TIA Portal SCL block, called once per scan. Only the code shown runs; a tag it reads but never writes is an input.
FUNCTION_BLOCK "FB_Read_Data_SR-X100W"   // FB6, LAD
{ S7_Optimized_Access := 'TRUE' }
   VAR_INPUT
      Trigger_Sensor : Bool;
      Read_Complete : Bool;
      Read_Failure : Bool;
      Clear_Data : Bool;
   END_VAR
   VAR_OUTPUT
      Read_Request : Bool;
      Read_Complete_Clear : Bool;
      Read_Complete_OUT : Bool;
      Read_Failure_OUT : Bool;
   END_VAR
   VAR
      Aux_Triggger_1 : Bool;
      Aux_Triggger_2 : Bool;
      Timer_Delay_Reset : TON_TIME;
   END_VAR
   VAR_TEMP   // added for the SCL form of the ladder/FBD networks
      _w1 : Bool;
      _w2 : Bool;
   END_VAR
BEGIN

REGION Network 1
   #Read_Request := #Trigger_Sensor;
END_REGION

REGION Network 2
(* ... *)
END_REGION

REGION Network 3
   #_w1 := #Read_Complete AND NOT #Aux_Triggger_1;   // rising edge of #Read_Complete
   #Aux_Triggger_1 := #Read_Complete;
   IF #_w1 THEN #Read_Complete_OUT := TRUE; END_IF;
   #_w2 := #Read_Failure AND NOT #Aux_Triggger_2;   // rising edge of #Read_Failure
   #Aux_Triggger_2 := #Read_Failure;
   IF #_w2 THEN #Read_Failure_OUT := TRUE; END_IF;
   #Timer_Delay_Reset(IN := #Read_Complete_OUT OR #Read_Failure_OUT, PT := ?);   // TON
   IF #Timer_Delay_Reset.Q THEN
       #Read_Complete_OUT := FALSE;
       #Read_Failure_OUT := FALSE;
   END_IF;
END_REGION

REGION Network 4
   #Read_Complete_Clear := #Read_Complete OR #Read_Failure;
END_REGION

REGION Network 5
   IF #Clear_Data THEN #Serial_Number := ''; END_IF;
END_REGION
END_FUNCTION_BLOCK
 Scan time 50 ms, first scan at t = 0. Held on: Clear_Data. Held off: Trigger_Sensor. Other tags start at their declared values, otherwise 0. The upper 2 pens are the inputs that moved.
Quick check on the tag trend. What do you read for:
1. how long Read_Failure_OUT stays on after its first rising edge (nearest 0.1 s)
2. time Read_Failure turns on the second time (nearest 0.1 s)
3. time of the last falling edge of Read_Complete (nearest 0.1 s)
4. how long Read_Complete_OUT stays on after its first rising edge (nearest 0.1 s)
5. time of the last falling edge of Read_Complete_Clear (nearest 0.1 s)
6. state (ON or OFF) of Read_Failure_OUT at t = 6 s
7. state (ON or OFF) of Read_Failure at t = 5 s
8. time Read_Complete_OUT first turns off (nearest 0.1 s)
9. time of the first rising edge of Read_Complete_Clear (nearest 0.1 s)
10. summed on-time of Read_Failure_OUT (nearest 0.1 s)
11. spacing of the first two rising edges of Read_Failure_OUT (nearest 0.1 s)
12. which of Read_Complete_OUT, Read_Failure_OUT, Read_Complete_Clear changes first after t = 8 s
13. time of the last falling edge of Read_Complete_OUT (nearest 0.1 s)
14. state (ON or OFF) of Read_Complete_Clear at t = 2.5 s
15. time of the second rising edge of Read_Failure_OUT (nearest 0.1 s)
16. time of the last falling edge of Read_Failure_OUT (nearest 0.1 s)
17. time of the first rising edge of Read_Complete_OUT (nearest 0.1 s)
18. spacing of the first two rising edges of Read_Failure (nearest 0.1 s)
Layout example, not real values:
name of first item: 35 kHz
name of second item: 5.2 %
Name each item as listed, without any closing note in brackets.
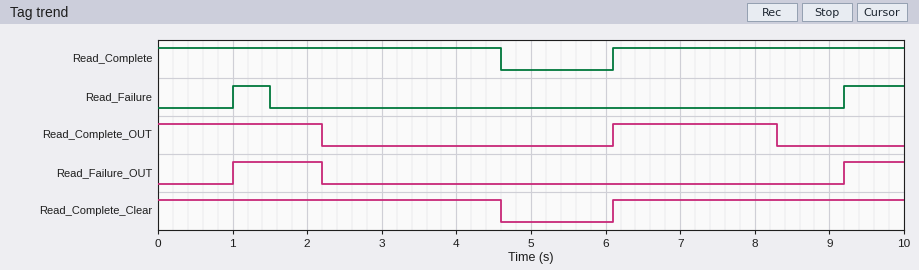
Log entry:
how long Read_Failure_OUT stays on after its first rising edge: 1.2 s
time Read_Failure turns on the second time: 9.2 s
time of the last falling edge of Read_Complete: 4.6 s
how long Read_Complete_OUT stays on after its first rising edge: 2.2 s
time of the last falling edge of Read_Complete_Clear: 4.6 s
state (ON or OFF) of Read_Failure_OUT at t = 6 s: OFF
state (ON or OFF) of Read_Failure at t = 5 s: OFF
time Read_Complete_OUT first turns off: 2.2 s
time of the first rising edge of Read_Complete_Clear: 6.1 s
summed on-time of Read_Failure_OUT: 2.0 s
spacing of the first two rising edges of Read_Failure_OUT: 8.2 s
which of Read_Complete_OUT, Read_Failure_OUT, Read_Complete_Clear changes first after t = 8 s: Read_Complete_OUT
time of the last falling edge of Read_Complete_OUT: 8.3 s
state (ON or OFF) of Read_Complete_Clear at t = 2.5 s: ON
time of the second rising edge of Read_Failure_OUT: 9.2 s
time of the last falling edge of Read_Failure_OUT: 2.2 s
time of the first rising edge of Read_Complete_OUT: 6.1 s
spacing of the first two rising edges of Read_Failure: 8.2 s
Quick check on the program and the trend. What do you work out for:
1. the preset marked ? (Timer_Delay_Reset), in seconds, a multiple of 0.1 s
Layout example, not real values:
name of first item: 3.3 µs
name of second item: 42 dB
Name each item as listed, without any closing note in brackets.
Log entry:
the preset marked ? (Timer_Delay_Reset), in seconds, a multiple of 0.1 s: 2.2 s
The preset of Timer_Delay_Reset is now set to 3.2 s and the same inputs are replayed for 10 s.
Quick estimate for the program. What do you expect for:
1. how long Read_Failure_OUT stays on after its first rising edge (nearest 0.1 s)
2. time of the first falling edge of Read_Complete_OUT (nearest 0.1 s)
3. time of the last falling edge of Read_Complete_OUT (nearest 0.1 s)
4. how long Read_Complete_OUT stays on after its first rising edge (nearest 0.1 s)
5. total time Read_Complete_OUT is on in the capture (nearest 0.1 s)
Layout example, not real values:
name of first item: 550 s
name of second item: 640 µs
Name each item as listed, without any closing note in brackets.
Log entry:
how long Read_Failure_OUT stays on after its first rising edge: 2.2 s
time of the first falling edge of Read_Complete_OUT: 3.2 s
time of the last falling edge of Read_Complete_OUT: 9.3 s
how long Read_Complete_OUT stays on after its first rising edge: 3.2 s
total time Read_Complete_OUT is on in the capture: 6.4 s
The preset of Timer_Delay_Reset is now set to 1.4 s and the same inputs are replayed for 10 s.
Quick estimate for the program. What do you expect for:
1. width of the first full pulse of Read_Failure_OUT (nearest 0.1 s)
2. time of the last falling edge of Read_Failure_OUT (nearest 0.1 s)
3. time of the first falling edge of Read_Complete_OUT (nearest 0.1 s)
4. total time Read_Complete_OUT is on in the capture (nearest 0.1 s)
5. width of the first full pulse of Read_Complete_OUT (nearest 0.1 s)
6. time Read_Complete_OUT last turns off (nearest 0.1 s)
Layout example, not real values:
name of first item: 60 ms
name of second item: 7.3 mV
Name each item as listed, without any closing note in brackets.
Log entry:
width of the first full pulse of Read_Failure_OUT: 0.4 s
time of the last falling edge of Read_Failure_OUT: 1.4 s
time of the first falling edge of Read_Complete_OUT: 1.4 s
total time Read_Complete_OUT is on in the capture: 2.8 s
width of the first full pulse of Read_Complete_OUT: 1.4 s
time Read_Complete_OUT last turns off: 7.5 s
